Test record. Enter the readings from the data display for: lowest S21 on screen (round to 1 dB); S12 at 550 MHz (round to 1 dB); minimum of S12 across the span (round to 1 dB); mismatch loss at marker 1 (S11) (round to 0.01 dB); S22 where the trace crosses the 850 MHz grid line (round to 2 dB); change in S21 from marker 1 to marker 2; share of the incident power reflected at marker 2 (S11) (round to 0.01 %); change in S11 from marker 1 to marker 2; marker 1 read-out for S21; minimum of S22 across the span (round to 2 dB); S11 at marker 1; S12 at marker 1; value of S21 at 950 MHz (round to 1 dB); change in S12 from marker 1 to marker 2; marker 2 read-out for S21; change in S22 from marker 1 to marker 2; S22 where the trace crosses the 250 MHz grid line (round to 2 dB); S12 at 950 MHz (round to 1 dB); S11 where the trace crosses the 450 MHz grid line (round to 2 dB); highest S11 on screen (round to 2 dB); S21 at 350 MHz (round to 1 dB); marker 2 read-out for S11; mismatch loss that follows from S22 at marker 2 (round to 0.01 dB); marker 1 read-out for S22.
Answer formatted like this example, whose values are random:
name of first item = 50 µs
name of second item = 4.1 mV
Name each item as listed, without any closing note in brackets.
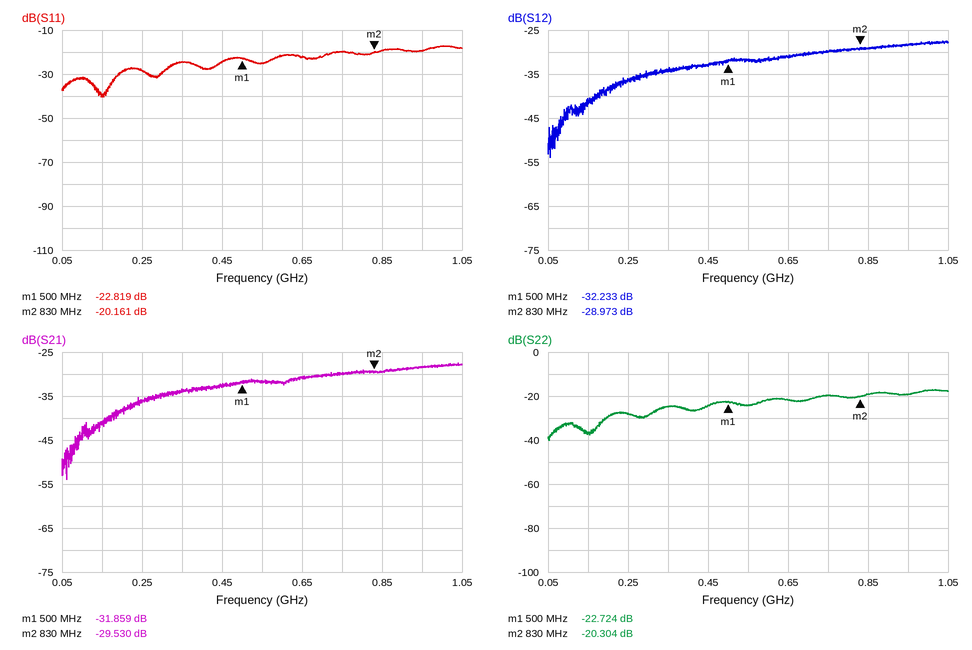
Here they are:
lowest S21 on screen = -54 dB
S12 at 550 MHz = -32 dB
minimum of S12 across the span = -54 dB
mismatch loss at marker 1 (S11) = 0.02 dB
S22 where the trace crosses the 850 MHz grid line = -20 dB
change in S21 from marker 1 to marker 2 = 2.329 dB
share of the incident power reflected at marker 2 (S11) = 0.96 %
change in S11 from marker 1 to marker 2 = 2.658 dB
marker 1 read-out for S21 = -31.859 dB
minimum of S22 across the span = -40 dB
S11 at marker 1 = -22.819 dB
S12 at marker 1 = -32.233 dB
value of S21 at 950 MHz = -28 dB
change in S12 from marker 1 to marker 2 = 3.260 dB
marker 2 read-out for S21 = -29.530 dB
change in S22 from marker 1 to marker 2 = 2.420 dB
S22 where the trace crosses the 250 MHz grid line = -28 dB
S12 at 950 MHz = -28 dB
S11 where the trace crosses the 450 MHz grid line = -24 dB
highest S11 on screen = -18 dB
S21 at 350 MHz = -34 dB
marker 2 read-out for S11 = -20.161 dB
mismatch loss that follows from S22 at marker 2 = 0.04 dB
marker 1 read-out for S22 = -22.724 dB
